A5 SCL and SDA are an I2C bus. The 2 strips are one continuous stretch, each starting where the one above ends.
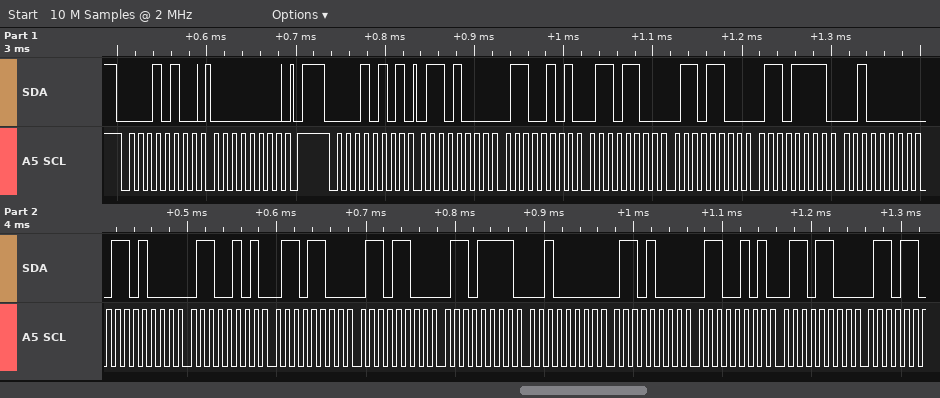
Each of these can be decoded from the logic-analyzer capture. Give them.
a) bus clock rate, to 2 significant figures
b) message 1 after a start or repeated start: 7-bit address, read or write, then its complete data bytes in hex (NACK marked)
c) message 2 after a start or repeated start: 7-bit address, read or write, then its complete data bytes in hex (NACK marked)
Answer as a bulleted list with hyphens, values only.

- 100 kHz
- 0x0A write: 00
- 0x0A read: 68 65 6C 6C 6F 20 68 65 6C 6C 6F 20 68 65 6C
